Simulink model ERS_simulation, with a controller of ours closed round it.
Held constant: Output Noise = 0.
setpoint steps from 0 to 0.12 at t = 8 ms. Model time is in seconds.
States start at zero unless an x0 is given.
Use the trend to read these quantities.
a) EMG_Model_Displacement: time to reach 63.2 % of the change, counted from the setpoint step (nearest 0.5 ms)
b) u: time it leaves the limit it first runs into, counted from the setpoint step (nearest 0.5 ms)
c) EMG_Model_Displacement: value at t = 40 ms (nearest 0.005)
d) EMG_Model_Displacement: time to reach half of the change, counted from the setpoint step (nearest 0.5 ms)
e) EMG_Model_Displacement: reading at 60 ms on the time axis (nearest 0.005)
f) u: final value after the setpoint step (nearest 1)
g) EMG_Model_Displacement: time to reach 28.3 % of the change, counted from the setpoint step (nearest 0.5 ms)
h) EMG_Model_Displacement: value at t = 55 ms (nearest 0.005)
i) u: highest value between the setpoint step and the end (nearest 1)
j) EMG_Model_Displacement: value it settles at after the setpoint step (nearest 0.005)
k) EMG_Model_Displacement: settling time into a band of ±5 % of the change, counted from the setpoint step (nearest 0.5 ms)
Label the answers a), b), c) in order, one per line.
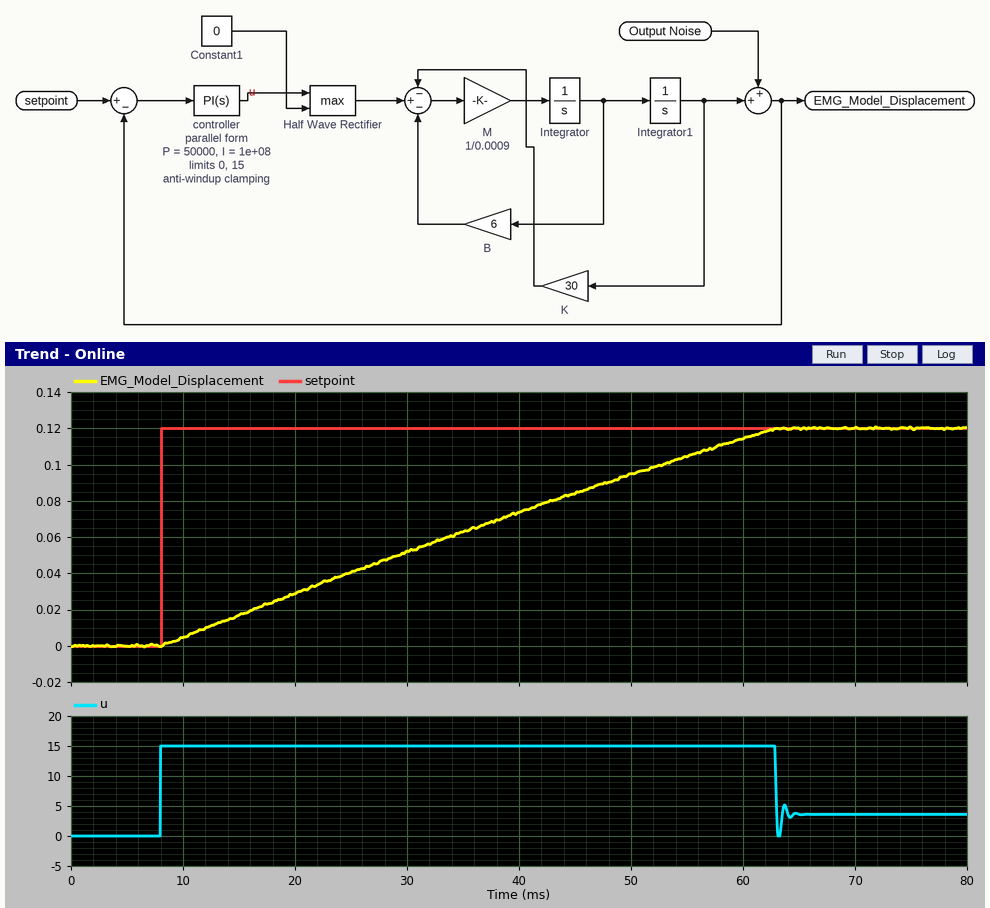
a) 33.0 ms
b) 55.0 ms
c) 0.075
d) 25.5 ms
e) 0.115
f) 4
g) 14.0 ms
h) 0.105
i) 15
j) 0.120
k) 52.0 ms
